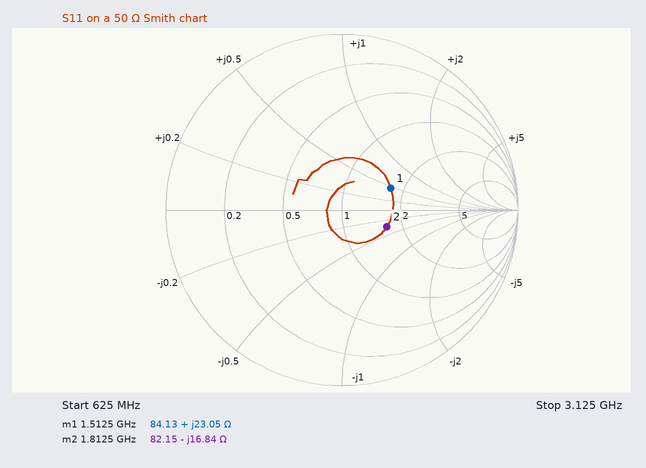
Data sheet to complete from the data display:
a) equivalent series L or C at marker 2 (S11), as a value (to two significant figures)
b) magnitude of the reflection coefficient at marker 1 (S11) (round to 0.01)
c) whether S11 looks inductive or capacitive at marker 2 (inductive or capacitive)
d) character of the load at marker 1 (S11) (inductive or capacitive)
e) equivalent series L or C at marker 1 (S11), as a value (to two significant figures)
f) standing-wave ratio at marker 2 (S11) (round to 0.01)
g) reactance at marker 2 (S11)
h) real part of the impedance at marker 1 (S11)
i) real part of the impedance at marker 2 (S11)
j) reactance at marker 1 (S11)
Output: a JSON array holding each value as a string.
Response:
["5.2 pF", "0.30", "capacitive", "inductive", "2.4 nH", "1.75", "-16.84 Ω", "84.13 Ω", "82.15 Ω", "+23.05 Ω"]
